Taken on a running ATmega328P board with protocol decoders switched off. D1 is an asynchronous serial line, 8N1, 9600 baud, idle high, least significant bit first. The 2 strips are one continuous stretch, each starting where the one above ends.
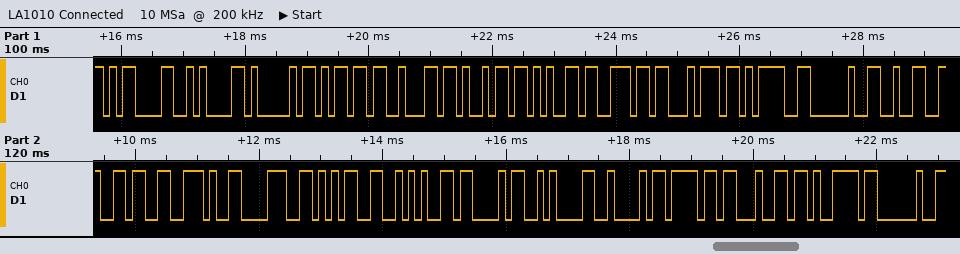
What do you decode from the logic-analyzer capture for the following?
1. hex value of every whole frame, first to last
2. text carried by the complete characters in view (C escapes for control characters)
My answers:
0D 0A 41 6D 62 69 65 6E 74 3D 20 32 36 2E 38 35 2A 43 0A 42 6F 64 79 20
"\r\nAmbient= 26.85*C\nBody "
